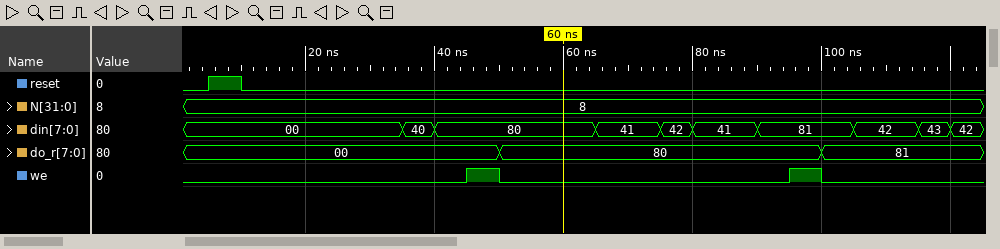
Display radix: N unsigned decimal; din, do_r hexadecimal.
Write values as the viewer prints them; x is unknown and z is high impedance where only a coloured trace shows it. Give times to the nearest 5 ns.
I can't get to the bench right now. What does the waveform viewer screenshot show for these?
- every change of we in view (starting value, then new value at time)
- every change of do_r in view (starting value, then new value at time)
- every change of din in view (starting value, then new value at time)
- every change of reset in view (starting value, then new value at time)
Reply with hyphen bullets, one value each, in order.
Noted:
- 0, 1 at 45 ns, 0 at 50 ns, 1 at 95 ns, 0 at 100 ns
- 00, 80 at 50 ns, 81 at 100 ns
- 00, 40 at 35 ns, 80 at 40 ns, 41 at 65 ns, 42 at 75 ns, 41 at 80 ns, 81 at 90 ns, 42 at 105 ns, 43 at 115 ns, 42 at 120 ns
- 0, 1 at 5 ns, 0 at 10 ns
